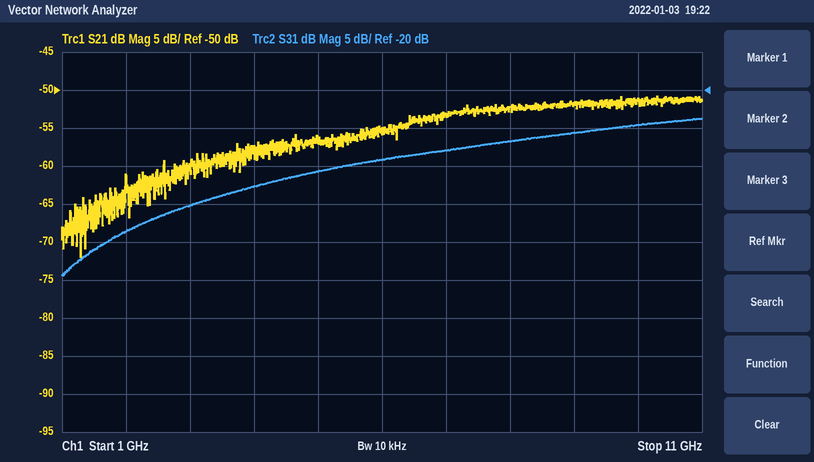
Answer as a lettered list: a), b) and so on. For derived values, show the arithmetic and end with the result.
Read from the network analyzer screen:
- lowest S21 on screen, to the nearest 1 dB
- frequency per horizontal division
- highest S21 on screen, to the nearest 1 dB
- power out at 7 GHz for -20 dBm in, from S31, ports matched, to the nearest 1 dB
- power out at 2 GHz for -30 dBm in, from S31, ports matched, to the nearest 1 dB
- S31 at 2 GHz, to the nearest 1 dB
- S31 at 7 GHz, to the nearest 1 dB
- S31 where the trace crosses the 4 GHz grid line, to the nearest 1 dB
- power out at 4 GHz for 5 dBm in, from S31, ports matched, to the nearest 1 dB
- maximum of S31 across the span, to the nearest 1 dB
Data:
a) -72 dB
b) 1 GHz
c) -51 dB
d) -20 dBm + (-28 dB) = -48 dBm
e) -30 dBm + (-39 dB) = -69 dBm
f) -39 dB
g) -28 dB
h) -33 dB
i) 5 dBm + (-33 dB) = -28 dBm
j) -24 dB
